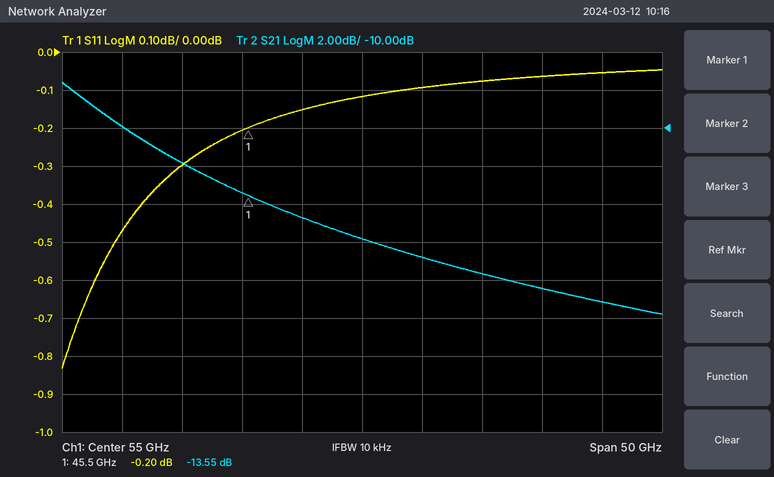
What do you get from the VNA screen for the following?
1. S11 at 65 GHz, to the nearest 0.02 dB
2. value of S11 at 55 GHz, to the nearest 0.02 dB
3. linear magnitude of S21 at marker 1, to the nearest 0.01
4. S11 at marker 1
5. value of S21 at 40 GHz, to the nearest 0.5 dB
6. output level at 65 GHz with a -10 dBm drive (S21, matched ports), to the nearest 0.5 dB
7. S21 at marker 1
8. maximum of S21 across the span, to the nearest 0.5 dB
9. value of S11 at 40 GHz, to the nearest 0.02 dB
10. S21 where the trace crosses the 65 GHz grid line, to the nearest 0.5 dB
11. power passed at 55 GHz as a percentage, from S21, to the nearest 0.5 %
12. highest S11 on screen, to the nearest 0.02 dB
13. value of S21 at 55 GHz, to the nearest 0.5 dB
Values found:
-0.08 dB
-0.12 dB
0.21
-0.20 dB
-12.0 dB
-27.5 dBm
-13.55 dB
-7.5 dB
-0.30 dB
-17.5 dB
2.5 %
-0.04 dB
-16.0 dB
